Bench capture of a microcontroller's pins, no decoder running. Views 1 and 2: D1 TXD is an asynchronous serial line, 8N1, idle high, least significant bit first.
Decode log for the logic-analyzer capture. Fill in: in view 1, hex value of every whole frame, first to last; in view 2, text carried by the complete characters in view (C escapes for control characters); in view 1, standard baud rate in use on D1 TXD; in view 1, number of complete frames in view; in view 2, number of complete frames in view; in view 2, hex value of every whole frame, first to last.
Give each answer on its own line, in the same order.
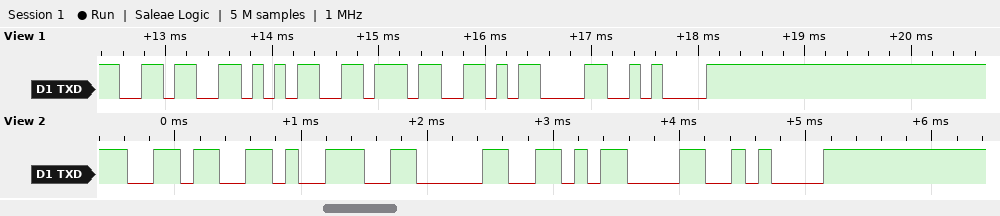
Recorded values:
36 35 37 0D 0A
"690\r\n"
9600 baud
5
5
0x36 0x39 0x30 0x0D 0x0A
